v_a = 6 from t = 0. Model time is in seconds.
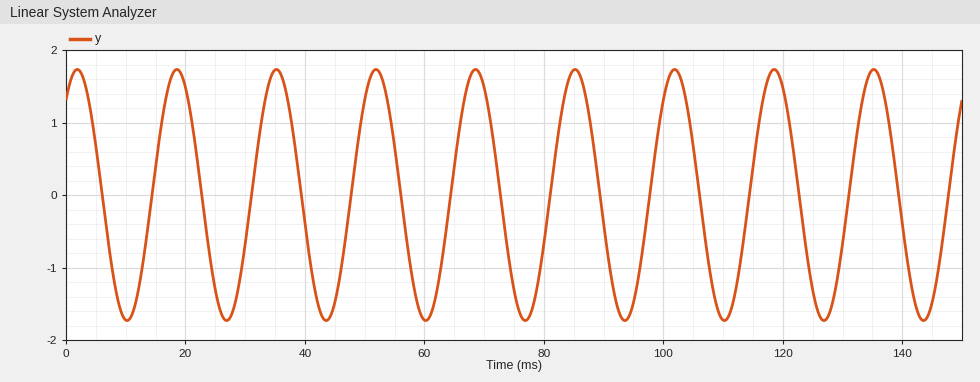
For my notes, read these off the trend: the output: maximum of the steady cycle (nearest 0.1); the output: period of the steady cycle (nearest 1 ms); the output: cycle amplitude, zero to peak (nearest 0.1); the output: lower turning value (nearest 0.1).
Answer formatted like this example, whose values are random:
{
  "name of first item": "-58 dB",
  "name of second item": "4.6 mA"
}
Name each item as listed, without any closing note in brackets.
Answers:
{
  "the output: maximum of the steady cycle": "1.7",
  "the output: period of the steady cycle": "17 ms",
  "the output: cycle amplitude, zero to peak": "1.7",
  "the output: lower turning value": "-1.7"
}
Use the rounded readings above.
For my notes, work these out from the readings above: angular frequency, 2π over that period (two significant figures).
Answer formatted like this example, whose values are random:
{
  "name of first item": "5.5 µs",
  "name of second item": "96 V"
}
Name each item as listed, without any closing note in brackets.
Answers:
{
  "angular frequency, 2π over that period": "0.37 rad/ms"
}
